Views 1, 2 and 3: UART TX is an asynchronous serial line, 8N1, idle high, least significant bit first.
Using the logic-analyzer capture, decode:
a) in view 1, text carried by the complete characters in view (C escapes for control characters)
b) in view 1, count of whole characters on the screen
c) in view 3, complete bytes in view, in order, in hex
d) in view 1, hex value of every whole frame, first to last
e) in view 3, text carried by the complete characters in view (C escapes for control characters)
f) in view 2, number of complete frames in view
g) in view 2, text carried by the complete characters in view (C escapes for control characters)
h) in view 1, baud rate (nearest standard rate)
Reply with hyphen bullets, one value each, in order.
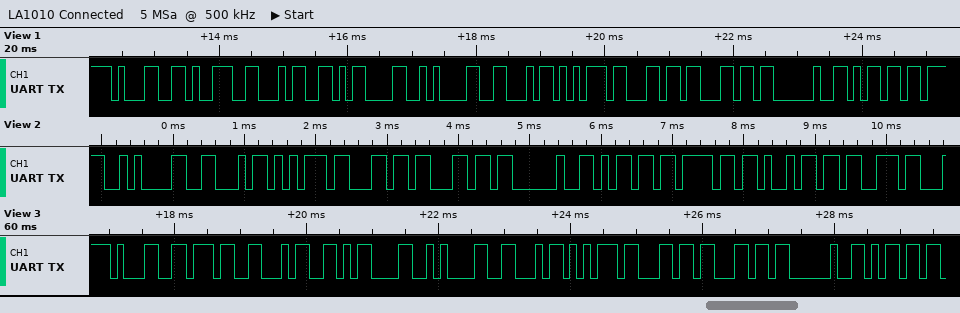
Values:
- "194\r\nFull m"
- 11
- 31 37 34 0D 0A 46 75 6C 6C 20 6D
- 31 39 34 0D 0A 46 75 6C 6C 20 6D
- "174\r\nFull m"
- 10
- "\nFull mois"
- 9600 baud
